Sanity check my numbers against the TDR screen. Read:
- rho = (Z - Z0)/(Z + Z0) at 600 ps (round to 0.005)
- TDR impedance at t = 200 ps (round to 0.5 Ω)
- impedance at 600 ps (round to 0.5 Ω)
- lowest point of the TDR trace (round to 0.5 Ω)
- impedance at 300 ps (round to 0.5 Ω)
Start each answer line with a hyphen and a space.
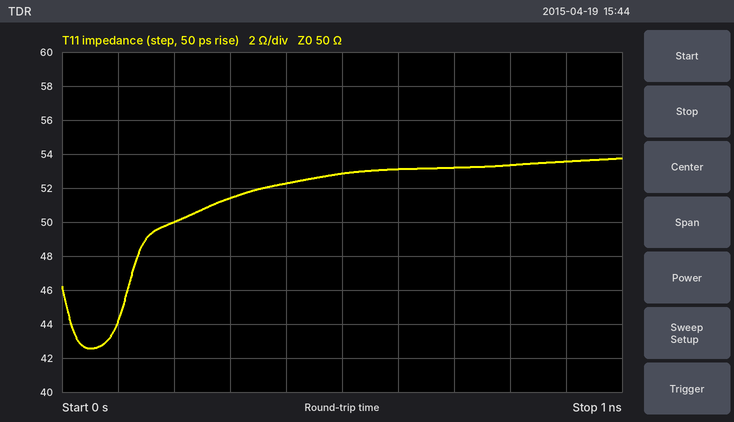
- +0.030
- 50.0 Ω
- 53.0 Ω
- 42.5 Ω
- 51.5 Ω
